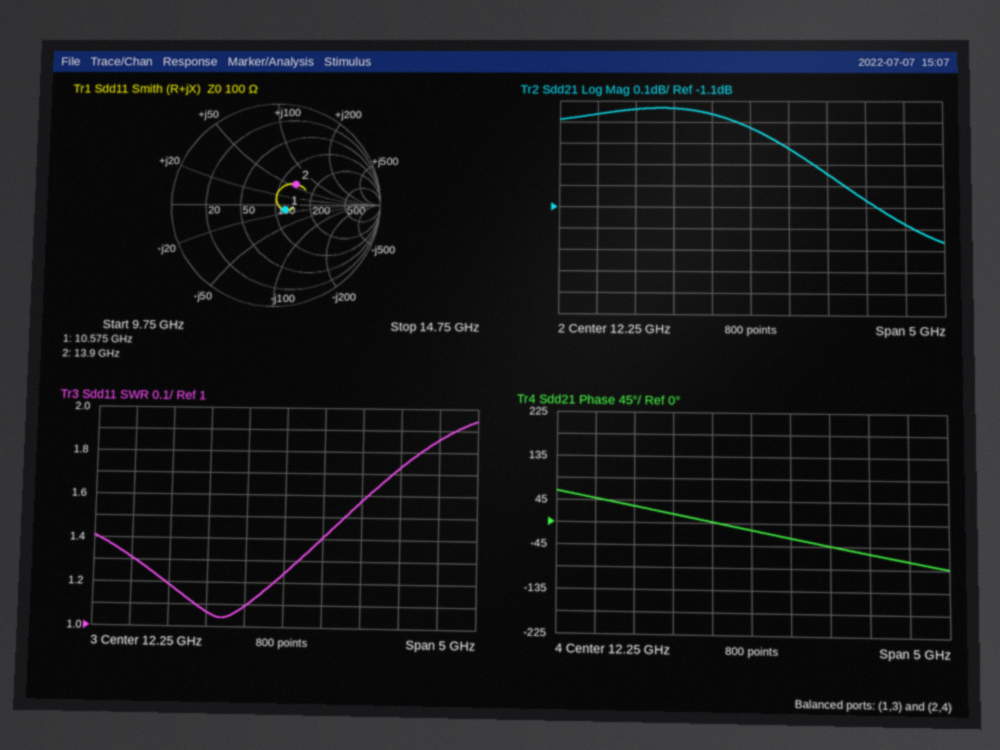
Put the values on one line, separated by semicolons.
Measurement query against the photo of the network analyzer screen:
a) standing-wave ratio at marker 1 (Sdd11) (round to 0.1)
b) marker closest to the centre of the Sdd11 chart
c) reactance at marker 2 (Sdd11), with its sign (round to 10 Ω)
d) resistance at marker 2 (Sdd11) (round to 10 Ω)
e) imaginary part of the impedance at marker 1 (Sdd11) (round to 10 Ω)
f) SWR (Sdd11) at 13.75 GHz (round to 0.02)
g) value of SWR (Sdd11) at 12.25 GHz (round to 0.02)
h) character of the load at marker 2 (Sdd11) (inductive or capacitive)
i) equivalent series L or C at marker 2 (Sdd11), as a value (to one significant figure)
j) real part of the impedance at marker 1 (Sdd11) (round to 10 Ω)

1.2; marker 1; +60 Ω; 130 Ω; -10 Ω; 1.72; 1.24; inductive; 700 pH; 120 Ω
